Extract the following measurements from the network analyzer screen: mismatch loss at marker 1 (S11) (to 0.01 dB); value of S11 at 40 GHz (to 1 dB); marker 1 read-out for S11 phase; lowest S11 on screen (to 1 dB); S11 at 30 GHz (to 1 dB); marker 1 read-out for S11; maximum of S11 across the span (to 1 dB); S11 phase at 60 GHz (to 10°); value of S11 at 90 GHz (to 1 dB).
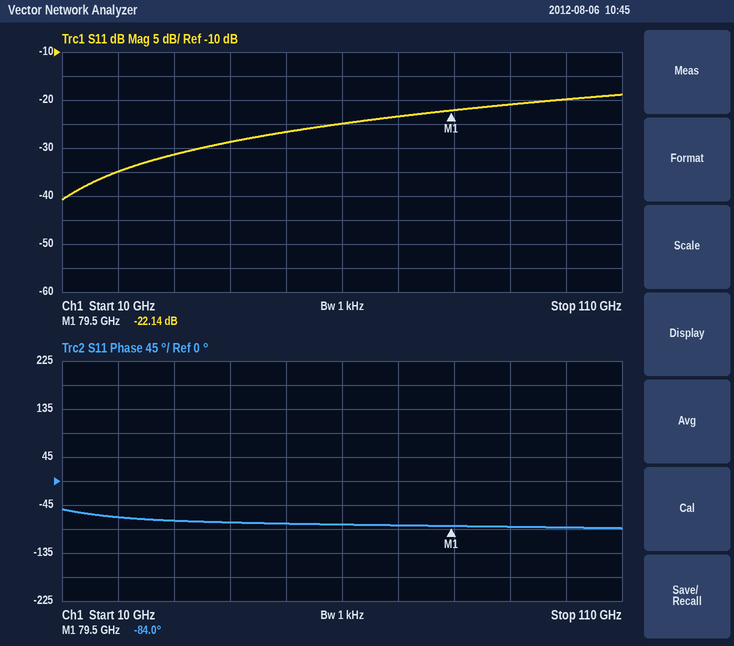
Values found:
0.03 dB
-29 dB
-84.0°
-41 dB
-31 dB
-22.14 dB
-19 dB
-80°
-21 dB
